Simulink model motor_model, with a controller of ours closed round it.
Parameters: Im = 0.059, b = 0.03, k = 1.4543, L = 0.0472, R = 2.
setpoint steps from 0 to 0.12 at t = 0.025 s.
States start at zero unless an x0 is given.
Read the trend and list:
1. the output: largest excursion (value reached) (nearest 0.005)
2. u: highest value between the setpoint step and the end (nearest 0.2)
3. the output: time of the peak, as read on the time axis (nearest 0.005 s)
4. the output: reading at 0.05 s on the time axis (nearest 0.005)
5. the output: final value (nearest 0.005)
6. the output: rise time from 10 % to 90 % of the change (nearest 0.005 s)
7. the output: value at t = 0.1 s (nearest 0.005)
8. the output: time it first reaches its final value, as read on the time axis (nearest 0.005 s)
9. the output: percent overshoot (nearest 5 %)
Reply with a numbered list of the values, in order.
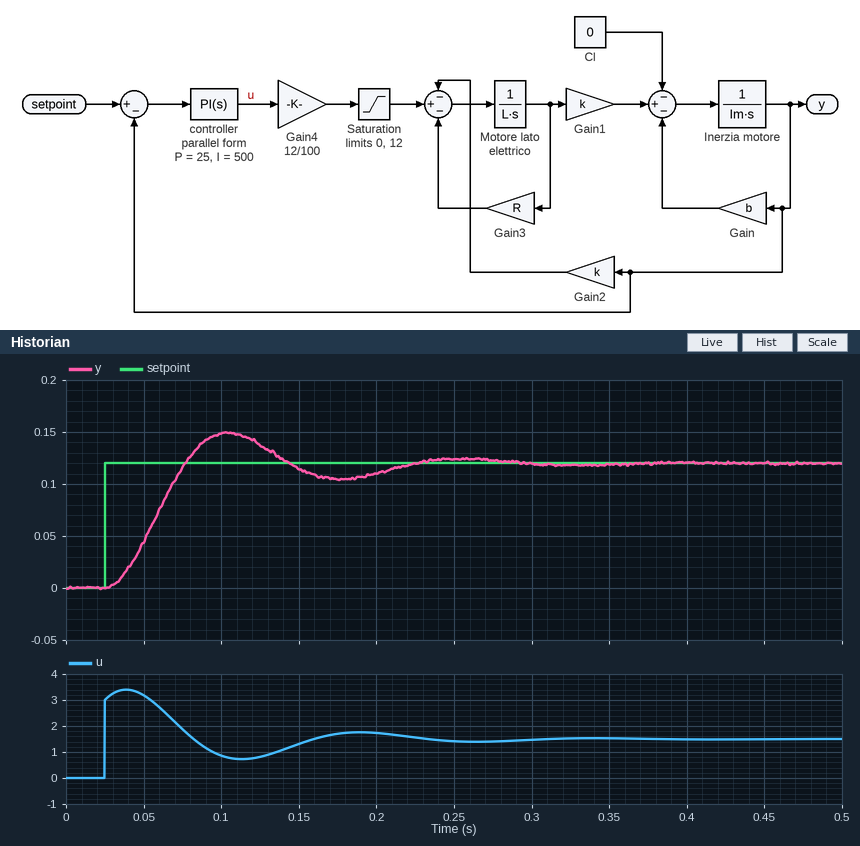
1. 0.150
2. 3.4
3. 0.105 s
4. 0.045
5. 0.120
6. 0.035 s
7. 0.150
8. 0.075 s
9. 25 %
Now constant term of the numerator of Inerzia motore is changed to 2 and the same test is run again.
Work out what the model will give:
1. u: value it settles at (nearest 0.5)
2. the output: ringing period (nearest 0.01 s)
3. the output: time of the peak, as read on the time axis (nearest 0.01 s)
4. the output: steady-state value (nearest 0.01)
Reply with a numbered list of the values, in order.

1. 1.5
2. 0.10 s
3. 0.08 s
4. 0.12
